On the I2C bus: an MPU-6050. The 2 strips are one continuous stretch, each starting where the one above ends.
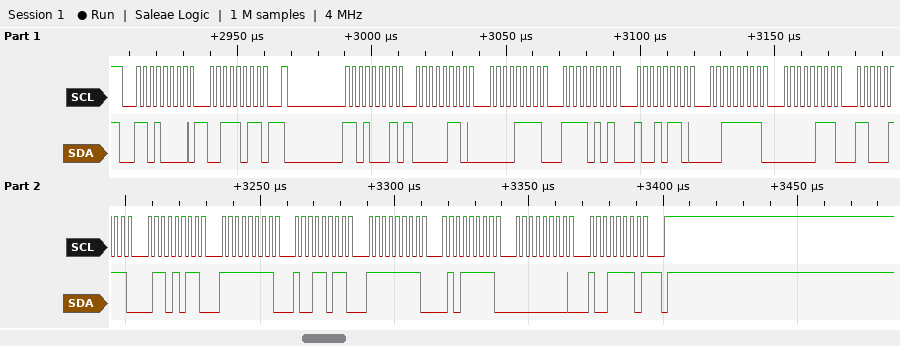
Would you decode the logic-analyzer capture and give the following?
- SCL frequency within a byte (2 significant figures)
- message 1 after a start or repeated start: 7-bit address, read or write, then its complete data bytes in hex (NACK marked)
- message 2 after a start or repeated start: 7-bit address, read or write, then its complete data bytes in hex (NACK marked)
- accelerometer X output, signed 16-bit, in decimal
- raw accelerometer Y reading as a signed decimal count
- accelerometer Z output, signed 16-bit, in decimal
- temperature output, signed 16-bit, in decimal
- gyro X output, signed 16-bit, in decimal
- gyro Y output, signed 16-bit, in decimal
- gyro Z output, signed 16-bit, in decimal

400 kHz
0x68 write: 3B
0x68 read: 06 0F F5 96 3F 07 C7 6B FF 9B FF 5F 00 9E NACK
1551
-2666
16135
-14485
-101
-161
158
